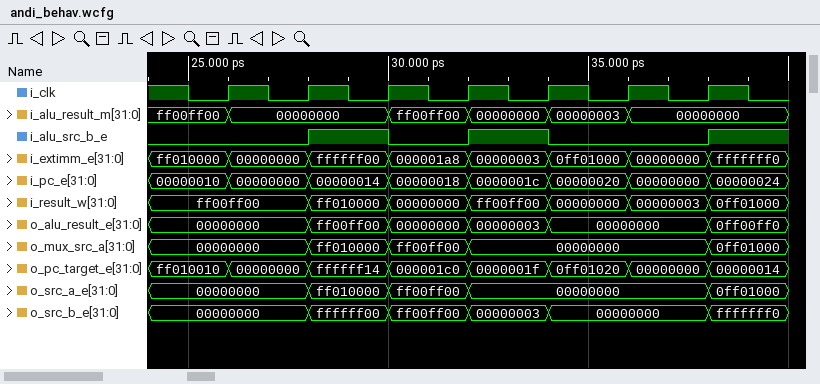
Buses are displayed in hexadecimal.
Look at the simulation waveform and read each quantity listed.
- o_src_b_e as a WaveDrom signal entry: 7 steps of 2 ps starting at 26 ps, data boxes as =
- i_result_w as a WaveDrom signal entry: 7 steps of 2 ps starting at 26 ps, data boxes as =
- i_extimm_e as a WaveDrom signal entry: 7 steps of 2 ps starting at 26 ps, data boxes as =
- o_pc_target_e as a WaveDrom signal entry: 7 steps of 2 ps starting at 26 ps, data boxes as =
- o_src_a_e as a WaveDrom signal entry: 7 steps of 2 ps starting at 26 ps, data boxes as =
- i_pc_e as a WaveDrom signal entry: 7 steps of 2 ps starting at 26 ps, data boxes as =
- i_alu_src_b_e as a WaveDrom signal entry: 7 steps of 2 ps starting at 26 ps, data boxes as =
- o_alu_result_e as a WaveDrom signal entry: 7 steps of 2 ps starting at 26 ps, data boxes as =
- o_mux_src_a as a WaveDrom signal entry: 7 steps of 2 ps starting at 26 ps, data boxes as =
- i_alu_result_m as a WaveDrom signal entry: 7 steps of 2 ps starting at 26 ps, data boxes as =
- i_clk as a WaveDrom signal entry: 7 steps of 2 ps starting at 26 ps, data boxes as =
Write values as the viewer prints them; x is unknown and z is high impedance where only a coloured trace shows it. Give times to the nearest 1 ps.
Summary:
{name: 'o_src_b_e', wave: '=====.=', data: '00000000 ffffff00 ff00ff00 00000003 00000000 fffffff0'}
{name: 'i_result_w', wave: '=======', data: 'ff00ff00 ff010000 00000000 ff00ff00 00000000 00000003 0ff01000'}
{name: 'i_extimm_e', wave: '=======', data: '00000000 ffffff00 000001a8 00000003 0ff01000 00000000 fffffff0'}
{name: 'o_pc_target_e', wave: '=======', data: '00000000 ffffff14 000001c0 0000001f 0ff01020 00000000 00000014'}
{name: 'o_src_a_e', wave: '====..=', data: '00000000 ff010000 ff00ff00 00000000 0ff01000'}
{name: 'i_pc_e', wave: '=======', data: '00000000 00000014 00000018 0000001c 00000020 00000000 00000024'}
{name: 'i_alu_src_b_e', wave: '01010.1'}
{name: 'o_alu_result_e', wave: '=====.=', data: '00000000 ff00ff00 00000000 00000003 00000000 0ff00ff0'}
{name: 'o_mux_src_a', wave: '====..=', data: '00000000 ff010000 ff00ff00 00000000 0ff01000'}
{name: 'i_alu_result_m', wave: '=.====.', data: '00000000 ff00ff00 00000000 00000003 00000000'}
{name: 'i_clk', wave: 'p......'}
